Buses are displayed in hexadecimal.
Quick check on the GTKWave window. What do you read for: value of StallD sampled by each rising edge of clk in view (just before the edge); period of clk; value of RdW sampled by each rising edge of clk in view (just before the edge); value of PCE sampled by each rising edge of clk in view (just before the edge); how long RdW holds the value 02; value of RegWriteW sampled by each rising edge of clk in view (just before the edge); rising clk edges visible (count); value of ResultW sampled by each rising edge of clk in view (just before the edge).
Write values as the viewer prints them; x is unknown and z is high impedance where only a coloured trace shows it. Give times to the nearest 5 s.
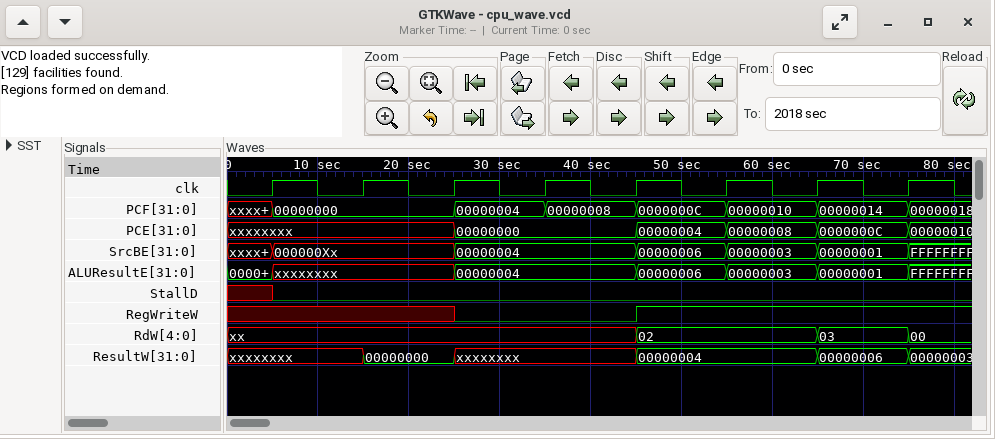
x 0 0 0 0 0 0 0
10 s
xx, xx, xx, xx, xx, 02, 02, 03
xxxxxxxx, xxxxxxxx, xxxxxxxx, 00000000, 00000000, 00000004, 00000008, 0000000C
20 s
x x x 0 0 1 1 1
8
xxxxxxxx, xxxxxxxx, 00000000, xxxxxxxx, xxxxxxxx, 00000004, 00000004, 00000006
